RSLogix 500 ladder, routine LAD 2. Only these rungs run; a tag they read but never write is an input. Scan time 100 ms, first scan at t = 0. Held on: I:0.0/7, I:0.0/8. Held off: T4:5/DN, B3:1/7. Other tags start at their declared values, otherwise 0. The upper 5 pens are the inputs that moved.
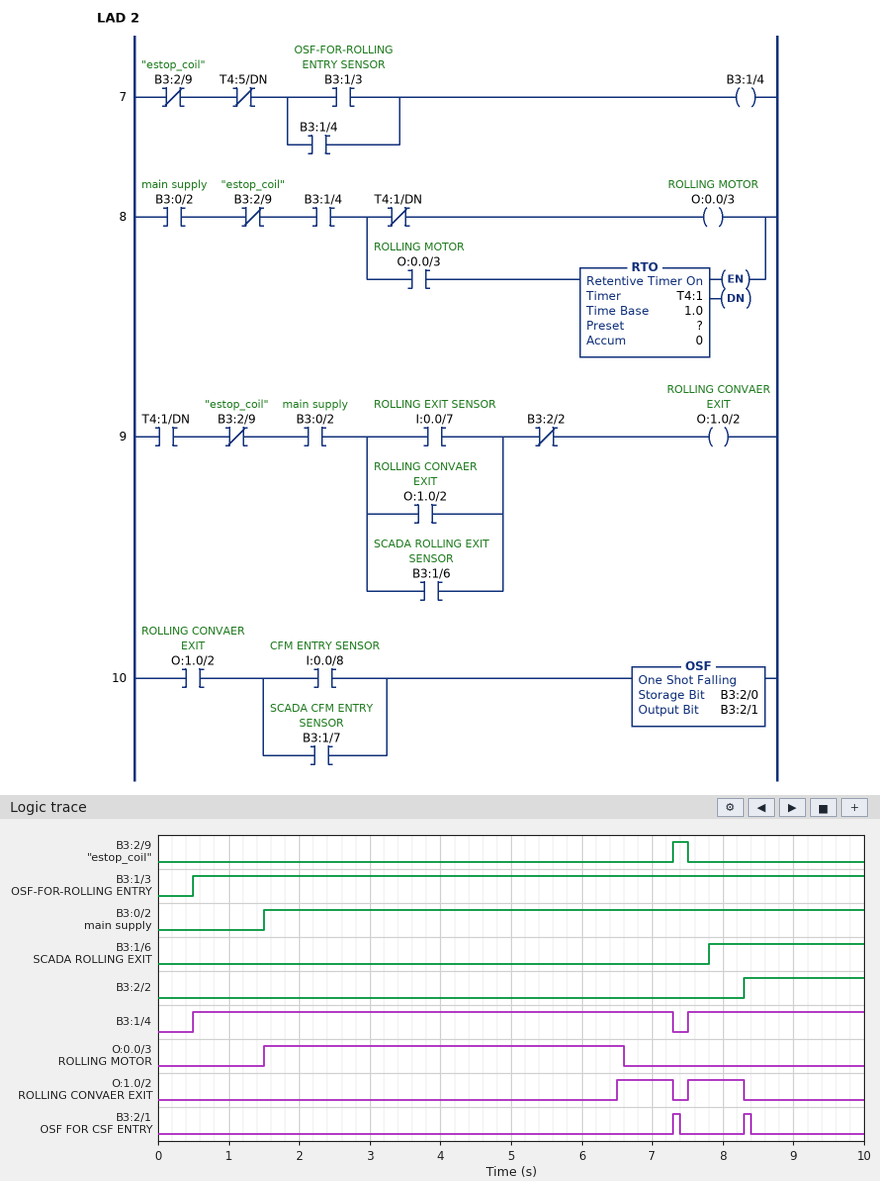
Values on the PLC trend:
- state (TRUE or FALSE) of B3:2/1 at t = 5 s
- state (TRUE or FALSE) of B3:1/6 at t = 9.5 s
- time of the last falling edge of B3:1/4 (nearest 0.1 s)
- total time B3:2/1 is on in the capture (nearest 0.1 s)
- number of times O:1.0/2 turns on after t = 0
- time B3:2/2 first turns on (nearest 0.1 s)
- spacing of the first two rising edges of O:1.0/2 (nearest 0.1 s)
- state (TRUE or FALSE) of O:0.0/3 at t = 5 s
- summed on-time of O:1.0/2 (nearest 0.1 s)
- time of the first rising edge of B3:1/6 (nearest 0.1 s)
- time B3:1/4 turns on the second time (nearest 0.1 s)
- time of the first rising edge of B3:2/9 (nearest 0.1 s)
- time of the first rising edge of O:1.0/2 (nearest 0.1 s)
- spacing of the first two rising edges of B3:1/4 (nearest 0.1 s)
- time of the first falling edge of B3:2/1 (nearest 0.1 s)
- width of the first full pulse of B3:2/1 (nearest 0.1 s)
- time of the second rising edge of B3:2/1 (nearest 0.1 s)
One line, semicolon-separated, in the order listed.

FALSE; TRUE; 7.3 s; 0.2 s; 2; 8.3 s; 1.0 s; TRUE; 1.6 s; 7.8 s; 7.5 s; 7.3 s; 6.5 s; 7.0 s; 7.4 s; 0.1 s; 8.3 s
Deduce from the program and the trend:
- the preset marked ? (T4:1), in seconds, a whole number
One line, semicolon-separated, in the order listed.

5 s
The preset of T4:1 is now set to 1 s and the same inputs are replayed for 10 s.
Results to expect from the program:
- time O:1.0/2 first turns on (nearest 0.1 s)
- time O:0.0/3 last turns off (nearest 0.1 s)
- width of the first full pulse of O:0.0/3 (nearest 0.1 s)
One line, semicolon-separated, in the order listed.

2.5 s; 2.6 s; 1.1 s
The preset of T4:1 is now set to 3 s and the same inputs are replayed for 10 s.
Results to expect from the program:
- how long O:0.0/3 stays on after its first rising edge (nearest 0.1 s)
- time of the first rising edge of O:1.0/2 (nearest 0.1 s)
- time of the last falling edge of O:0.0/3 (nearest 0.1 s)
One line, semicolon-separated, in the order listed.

3.1 s; 4.5 s; 4.6 s
